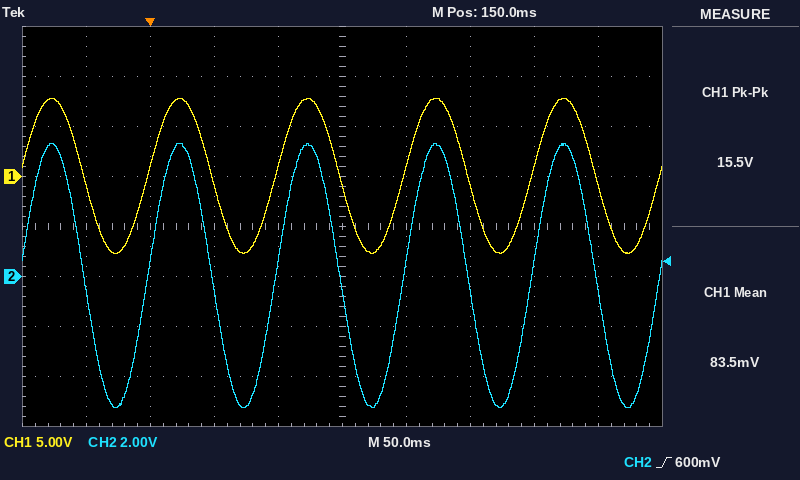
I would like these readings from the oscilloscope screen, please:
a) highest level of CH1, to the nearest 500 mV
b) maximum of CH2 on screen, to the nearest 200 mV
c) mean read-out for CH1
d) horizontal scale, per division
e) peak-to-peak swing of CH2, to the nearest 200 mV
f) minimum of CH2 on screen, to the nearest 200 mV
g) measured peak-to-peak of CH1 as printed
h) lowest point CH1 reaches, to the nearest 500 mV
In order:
8.0 V
5.4 V
83.5 mV
50 ms
10.6 V
-5.2 V
15.5 V
-7.5 V
